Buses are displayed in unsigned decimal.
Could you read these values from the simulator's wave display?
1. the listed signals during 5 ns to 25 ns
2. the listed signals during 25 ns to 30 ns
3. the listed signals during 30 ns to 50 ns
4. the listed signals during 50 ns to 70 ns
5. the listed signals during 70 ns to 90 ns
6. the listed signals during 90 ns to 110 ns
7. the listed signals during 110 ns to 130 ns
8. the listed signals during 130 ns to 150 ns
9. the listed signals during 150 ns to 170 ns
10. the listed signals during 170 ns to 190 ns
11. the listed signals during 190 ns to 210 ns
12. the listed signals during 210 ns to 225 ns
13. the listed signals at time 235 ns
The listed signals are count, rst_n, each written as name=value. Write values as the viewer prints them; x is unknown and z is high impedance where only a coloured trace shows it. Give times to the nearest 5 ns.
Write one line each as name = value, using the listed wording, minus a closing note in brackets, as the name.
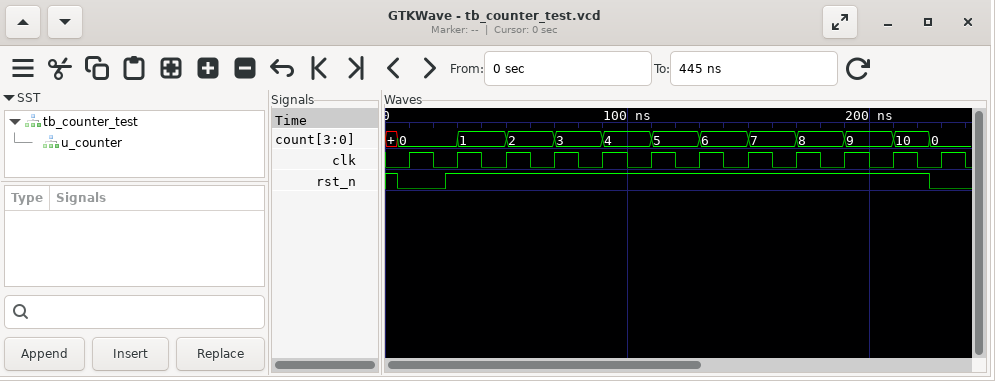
the listed signals during 5 ns to 25 ns = count=0, rst_n=0
the listed signals during 25 ns to 30 ns = count=0, rst_n=1
the listed signals during 30 ns to 50 ns = count=1, rst_n=1
the listed signals during 50 ns to 70 ns = count=2, rst_n=1
the listed signals during 70 ns to 90 ns = count=3, rst_n=1
the listed signals during 90 ns to 110 ns = count=4, rst_n=1
the listed signals during 110 ns to 130 ns = count=5, rst_n=1
the listed signals during 130 ns to 150 ns = count=6, rst_n=1
the listed signals during 150 ns to 170 ns = count=7, rst_n=1
the listed signals during 170 ns to 190 ns = count=8, rst_n=1
the listed signals during 190 ns to 210 ns = count=9, rst_n=1
the listed signals during 210 ns to 225 ns = count=10, rst_n=1
the listed signals at time 235 ns = count=0, rst_n=0
